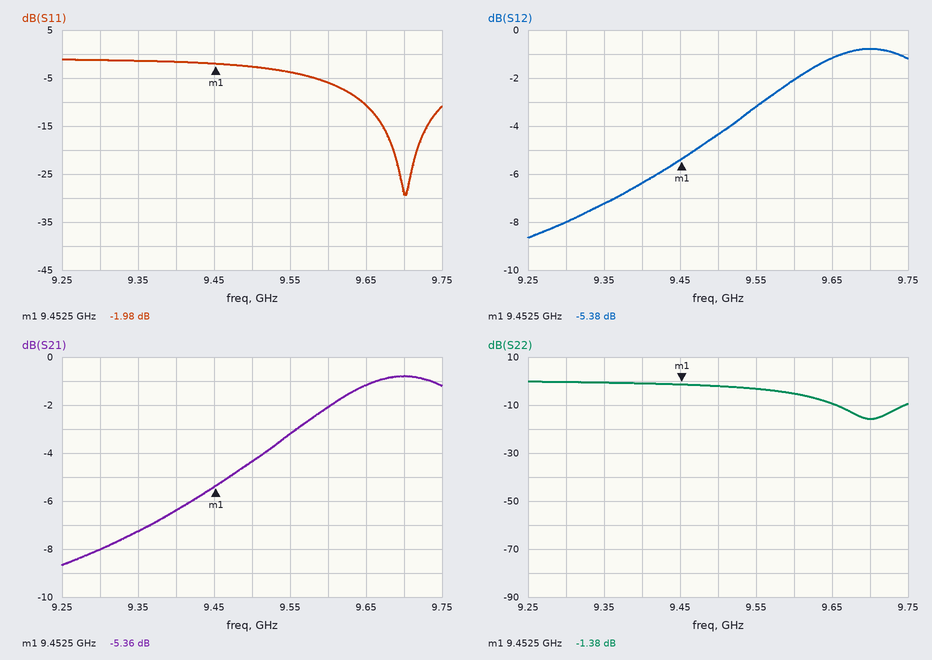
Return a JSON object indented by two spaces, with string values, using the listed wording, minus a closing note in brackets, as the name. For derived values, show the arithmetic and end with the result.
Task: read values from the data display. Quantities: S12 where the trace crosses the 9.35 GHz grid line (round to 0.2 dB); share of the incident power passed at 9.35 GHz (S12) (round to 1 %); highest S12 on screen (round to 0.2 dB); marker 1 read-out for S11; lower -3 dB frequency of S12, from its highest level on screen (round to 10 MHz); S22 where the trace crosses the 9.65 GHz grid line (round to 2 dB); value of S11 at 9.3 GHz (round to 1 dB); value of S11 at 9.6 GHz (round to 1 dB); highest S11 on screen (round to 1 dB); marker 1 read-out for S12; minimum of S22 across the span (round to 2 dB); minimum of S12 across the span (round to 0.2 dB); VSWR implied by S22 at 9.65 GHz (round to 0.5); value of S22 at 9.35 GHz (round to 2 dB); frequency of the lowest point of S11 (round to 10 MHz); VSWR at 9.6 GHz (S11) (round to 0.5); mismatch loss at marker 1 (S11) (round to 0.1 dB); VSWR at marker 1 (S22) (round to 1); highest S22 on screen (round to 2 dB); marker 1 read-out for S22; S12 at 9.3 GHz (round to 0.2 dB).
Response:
{
  "S12 where the trace crosses the 9.35 GHz grid line": "-7.2 dB",
  "share of the incident power passed at 9.35 GHz (S12)": "10^(-7.2/10) ≈ 19 %",
  "highest S12 on screen": "-0.8 dB",
  "marker 1 read-out for S11": "-1.98 dB",
  "lower -3 dB frequency of S12, from its highest level on screen": "9.53 GHz",
  "S22 where the trace crosses the 9.65 GHz grid line": "-10 dB",
  "value of S11 at 9.3 GHz": "-1 dB",
  "value of S11 at 9.6 GHz": "-6 dB",
  "highest S11 on screen": "-1 dB",
  "marker 1 read-out for S12": "-5.38 dB",
  "minimum of S22 across the span": "-16 dB",
  "minimum of S12 across the span": "-8.6 dB",
  "VSWR implied by S22 at 9.65 GHz": "|Γ| = 10^(-10/20) = 0.3162; VSWR = (1 + 0.3162)/(1 − 0.3162) ≈ 1.92, so 2.0 to the nearest 0.5",
  "value of S22 at 9.35 GHz": "0 dB",
  "frequency of the lowest point of S11": "9.70 GHz",
  "VSWR at 9.6 GHz (S11)": "|Γ| = 10^(-6/20) = 0.5012; VSWR = (1 + 0.5012)/(1 − 0.5012) ≈ 3.0",
  "mismatch loss at marker 1 (S11)": "−10 log10(1 − 10^(-1.98/10)) ≈ 4.4 dB",
  "VSWR at marker 1 (S22)": "(1 + 0.8531)/(1 − 0.8531) ≈ 13",
  "highest S22 on screen": "0 dB",
  "marker 1 read-out for S22": "-1.38 dB",
  "S12 at 9.3 GHz": "-8.0 dB"
}
